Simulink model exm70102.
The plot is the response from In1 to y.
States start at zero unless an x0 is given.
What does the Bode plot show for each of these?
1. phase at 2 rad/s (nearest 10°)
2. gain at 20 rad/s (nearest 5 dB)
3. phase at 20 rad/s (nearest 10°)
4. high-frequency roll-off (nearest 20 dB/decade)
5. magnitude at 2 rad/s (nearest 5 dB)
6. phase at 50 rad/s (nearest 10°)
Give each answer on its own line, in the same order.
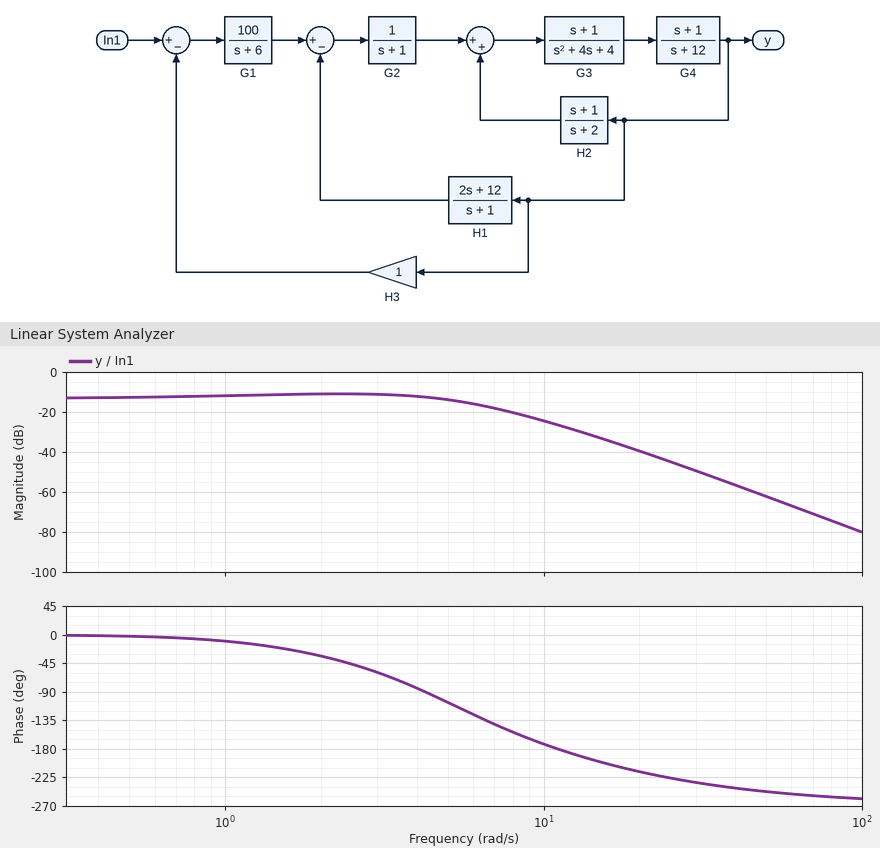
-30°
-40 dB
-220°
-60 dB/decade
-10 dB
-250°
